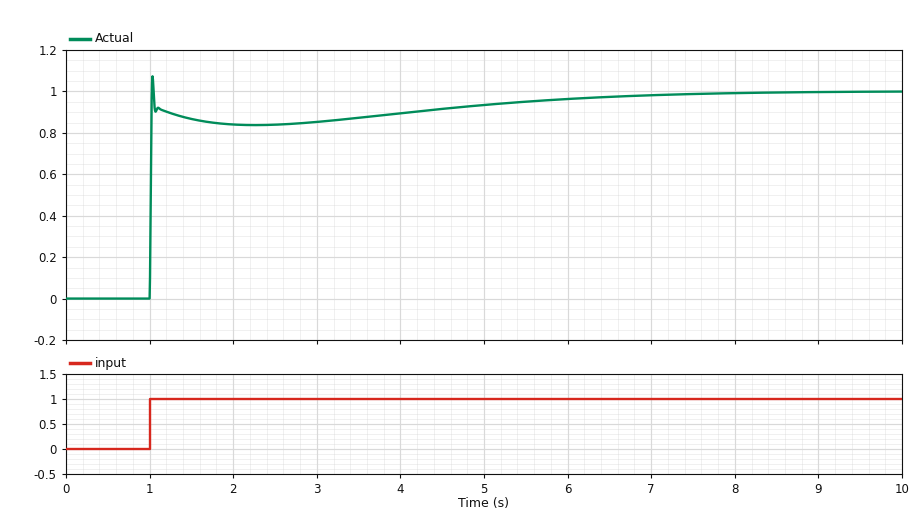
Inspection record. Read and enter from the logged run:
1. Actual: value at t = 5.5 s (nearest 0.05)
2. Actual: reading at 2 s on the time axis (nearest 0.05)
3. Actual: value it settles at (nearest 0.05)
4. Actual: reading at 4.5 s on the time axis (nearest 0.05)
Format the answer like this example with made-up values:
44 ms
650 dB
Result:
0.95
0.85
1.00
0.90
